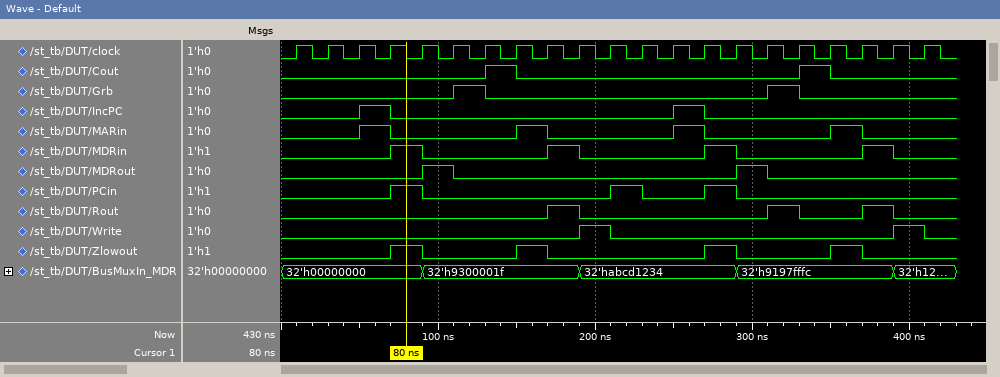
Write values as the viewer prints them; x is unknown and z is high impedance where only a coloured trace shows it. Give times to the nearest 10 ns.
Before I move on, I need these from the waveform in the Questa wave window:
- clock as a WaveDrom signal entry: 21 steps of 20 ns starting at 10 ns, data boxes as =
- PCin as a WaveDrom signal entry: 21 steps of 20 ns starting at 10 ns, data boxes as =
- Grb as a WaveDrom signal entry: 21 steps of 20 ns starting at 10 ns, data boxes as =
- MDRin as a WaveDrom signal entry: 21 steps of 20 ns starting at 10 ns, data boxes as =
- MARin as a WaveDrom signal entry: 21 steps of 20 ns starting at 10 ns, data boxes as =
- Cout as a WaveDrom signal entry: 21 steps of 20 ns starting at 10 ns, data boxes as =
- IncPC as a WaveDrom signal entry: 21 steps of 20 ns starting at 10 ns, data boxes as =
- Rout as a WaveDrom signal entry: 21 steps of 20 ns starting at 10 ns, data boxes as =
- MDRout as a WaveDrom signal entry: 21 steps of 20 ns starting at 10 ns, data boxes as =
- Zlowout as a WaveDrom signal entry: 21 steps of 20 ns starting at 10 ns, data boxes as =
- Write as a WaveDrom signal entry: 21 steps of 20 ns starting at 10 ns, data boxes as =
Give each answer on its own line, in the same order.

{name: 'clock', wave: 'p....................'}
{name: 'PCin', wave: '0..10.....10.10......'}
{name: 'Grb', wave: '0....10........10....'}
{name: 'MDRin', wave: '0..10...10...10...10.'}
{name: 'MARin', wave: '0.10...10...10...10..'}
{name: 'Cout', wave: '0.....10........10...'}
{name: 'IncPC', wave: '0.10........10.......'}
{name: 'Rout', wave: '0.......10.....10.10.'}
{name: 'MDRout', wave: '0...10........10.....'}
{name: 'Zlowout', wave: '0..10..10....10..10..'}
{name: 'Write', wave: '0........10........10'}
